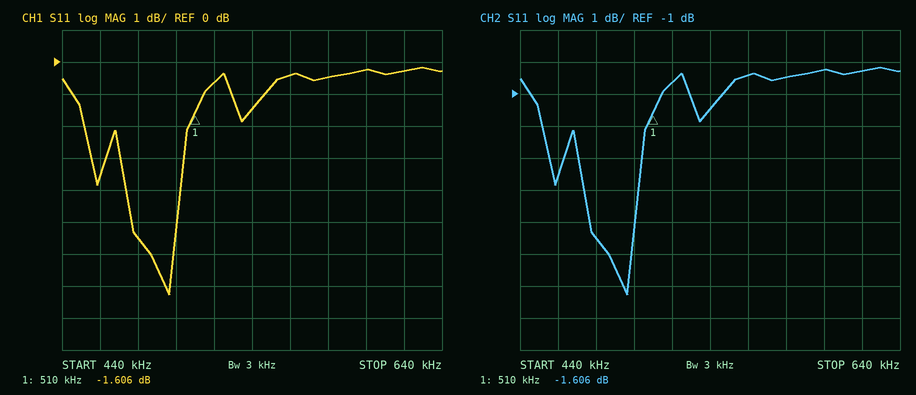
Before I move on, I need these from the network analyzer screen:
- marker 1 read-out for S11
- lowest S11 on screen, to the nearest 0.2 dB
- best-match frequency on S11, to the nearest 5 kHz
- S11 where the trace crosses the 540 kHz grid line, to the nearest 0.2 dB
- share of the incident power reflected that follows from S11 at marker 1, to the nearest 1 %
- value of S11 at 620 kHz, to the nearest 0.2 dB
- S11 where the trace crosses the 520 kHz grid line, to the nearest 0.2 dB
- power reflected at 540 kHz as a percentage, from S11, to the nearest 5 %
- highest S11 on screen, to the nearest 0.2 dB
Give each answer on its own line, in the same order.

-1.606 dB
-7.2 dB
495 kHz
-1.4 dB
69 %
-0.2 dB
-0.6 dB
70 %
-0.2 dB
